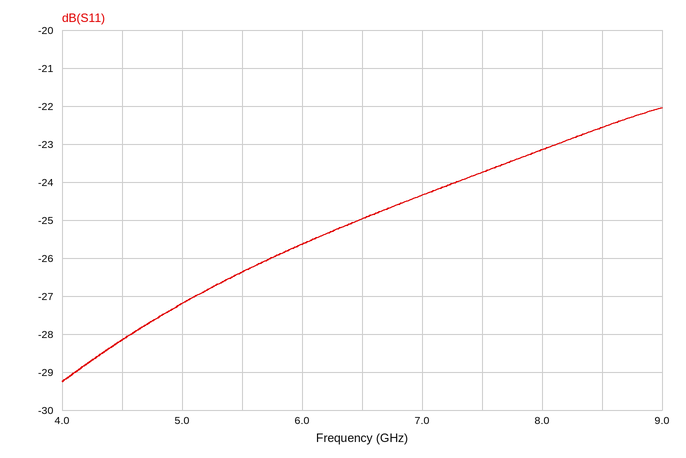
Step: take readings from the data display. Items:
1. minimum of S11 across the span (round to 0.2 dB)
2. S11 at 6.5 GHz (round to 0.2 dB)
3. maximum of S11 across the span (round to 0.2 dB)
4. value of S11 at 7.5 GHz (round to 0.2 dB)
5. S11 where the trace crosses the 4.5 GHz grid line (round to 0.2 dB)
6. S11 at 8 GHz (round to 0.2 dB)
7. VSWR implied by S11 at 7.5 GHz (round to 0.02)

-29.2 dB
-25.0 dB
-22.0 dB
-23.8 dB
-28.2 dB
-23.2 dB
1.14
